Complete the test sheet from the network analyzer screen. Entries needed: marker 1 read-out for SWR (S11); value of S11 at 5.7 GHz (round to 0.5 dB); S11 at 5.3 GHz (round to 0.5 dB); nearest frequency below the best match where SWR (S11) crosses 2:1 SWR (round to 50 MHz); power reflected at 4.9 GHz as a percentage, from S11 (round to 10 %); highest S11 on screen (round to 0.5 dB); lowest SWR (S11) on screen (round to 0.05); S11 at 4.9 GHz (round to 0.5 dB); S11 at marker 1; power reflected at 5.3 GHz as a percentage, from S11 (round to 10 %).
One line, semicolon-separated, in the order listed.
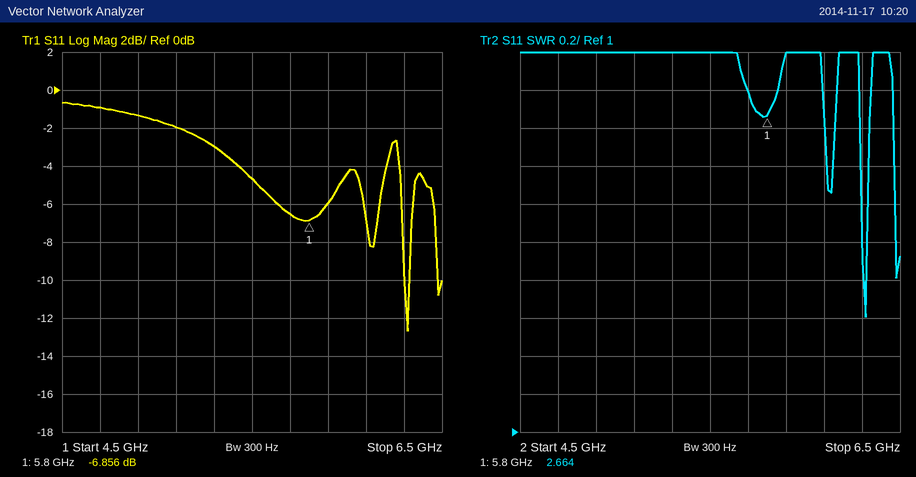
2.664; -6.5 dB; -3.0 dB; 6.30 GHz; 70 %; -0.5 dB; 1.60; -1.5 dB; -6.856 dB; 50 %
